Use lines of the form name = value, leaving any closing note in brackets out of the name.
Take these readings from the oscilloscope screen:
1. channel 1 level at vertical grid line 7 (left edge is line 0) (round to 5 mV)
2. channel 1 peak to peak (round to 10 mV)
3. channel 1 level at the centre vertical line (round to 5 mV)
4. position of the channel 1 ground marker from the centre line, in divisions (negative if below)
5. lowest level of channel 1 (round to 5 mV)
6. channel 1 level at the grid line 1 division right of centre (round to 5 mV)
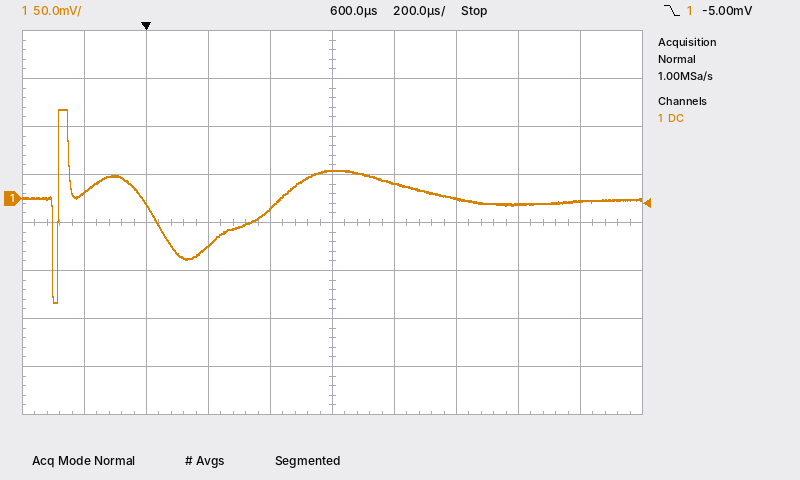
channel 1 level at vertical grid line 7 (left edge is line 0) = 0 mV
channel 1 peak to peak = 200 mV
channel 1 level at the centre vertical line = 30 mV
position of the channel 1 ground marker from the centre line, in divisions = +0.5 div
lowest level of channel 1 = -110 mV
channel 1 level at the grid line 1 division right of centre = 15 mV
